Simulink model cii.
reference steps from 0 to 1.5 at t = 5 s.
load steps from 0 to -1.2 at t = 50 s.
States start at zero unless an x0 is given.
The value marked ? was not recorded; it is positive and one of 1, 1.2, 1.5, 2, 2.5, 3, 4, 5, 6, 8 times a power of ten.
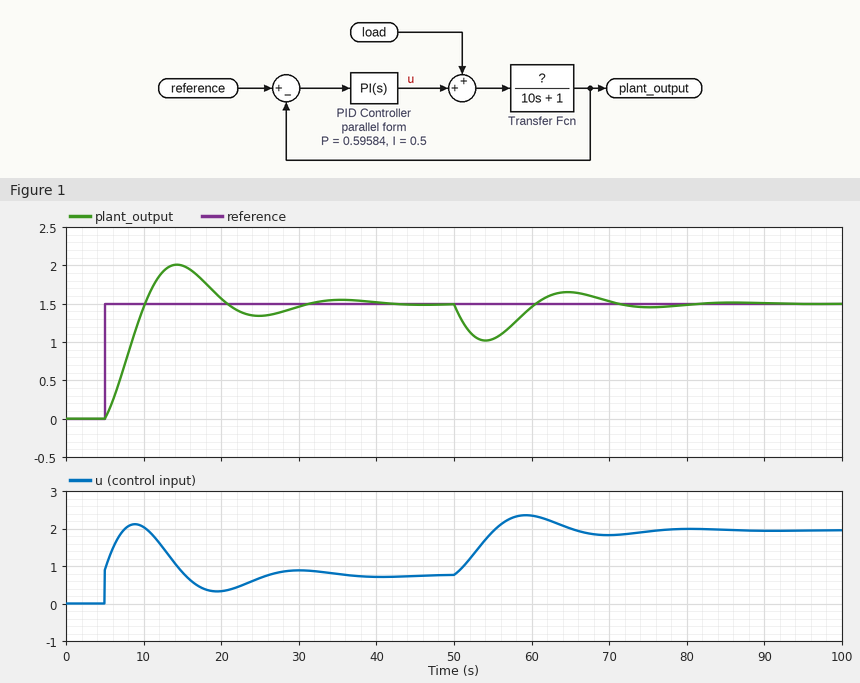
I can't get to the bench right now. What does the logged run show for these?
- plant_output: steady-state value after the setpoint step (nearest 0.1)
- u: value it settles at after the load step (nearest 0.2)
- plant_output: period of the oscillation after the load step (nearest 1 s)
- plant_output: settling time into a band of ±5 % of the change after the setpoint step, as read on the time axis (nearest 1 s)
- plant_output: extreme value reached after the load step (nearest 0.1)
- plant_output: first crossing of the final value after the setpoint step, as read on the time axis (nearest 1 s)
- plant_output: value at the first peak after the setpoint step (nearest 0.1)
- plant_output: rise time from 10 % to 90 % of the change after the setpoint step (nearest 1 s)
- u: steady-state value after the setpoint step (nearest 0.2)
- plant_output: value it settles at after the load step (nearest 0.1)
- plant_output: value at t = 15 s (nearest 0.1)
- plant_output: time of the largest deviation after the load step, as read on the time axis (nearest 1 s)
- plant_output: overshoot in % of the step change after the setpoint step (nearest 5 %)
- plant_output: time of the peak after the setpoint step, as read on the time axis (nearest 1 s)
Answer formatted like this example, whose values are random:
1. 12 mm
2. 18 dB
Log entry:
1. 1.5
2. 2.0
3. 21 s
4. 29 s
5. 1.0
6. 10 s
7. 2.0
8. 4 s
9. 0.8
10. 1.5
11. 2.0
12. 54 s
13. 35 %
14. 14 s
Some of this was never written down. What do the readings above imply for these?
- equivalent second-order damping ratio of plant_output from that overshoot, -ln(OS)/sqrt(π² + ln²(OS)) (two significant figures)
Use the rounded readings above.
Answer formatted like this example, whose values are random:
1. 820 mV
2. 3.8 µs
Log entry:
1. 0.32
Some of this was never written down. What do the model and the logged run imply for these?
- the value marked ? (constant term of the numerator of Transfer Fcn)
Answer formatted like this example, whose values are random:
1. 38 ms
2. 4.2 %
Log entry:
1. 2
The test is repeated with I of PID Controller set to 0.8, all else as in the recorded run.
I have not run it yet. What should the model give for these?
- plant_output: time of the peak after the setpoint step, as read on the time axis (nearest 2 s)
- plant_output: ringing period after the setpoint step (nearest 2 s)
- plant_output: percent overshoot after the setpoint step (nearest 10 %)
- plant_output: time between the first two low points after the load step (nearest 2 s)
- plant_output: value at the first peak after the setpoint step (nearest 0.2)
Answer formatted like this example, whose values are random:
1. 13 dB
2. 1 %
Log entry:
1. 12 s
2. 16 s
3. 40 %
4. 16 s
5. 2.2
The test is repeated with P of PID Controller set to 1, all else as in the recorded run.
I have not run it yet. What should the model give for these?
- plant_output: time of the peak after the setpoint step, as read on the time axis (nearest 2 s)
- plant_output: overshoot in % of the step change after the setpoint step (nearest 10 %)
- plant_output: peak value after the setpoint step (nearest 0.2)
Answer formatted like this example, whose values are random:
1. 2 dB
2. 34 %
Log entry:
1. 14 s
2. 20 %
3. 1.8
